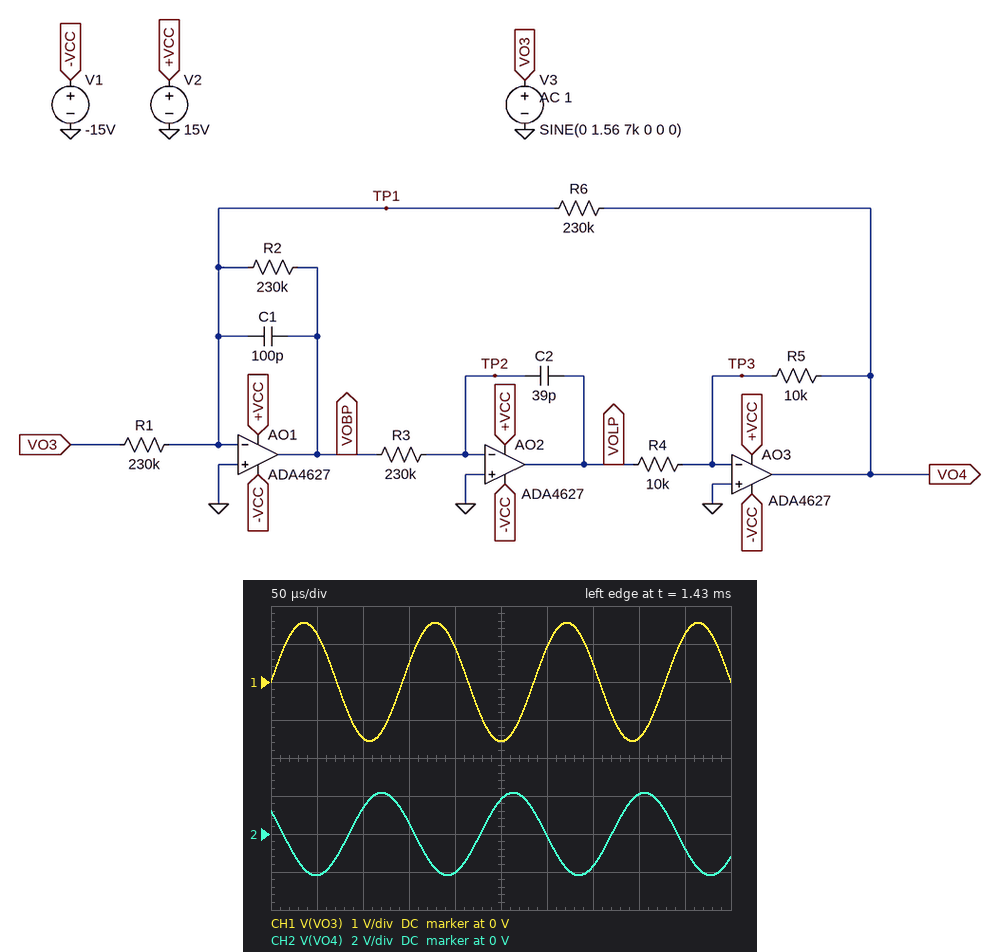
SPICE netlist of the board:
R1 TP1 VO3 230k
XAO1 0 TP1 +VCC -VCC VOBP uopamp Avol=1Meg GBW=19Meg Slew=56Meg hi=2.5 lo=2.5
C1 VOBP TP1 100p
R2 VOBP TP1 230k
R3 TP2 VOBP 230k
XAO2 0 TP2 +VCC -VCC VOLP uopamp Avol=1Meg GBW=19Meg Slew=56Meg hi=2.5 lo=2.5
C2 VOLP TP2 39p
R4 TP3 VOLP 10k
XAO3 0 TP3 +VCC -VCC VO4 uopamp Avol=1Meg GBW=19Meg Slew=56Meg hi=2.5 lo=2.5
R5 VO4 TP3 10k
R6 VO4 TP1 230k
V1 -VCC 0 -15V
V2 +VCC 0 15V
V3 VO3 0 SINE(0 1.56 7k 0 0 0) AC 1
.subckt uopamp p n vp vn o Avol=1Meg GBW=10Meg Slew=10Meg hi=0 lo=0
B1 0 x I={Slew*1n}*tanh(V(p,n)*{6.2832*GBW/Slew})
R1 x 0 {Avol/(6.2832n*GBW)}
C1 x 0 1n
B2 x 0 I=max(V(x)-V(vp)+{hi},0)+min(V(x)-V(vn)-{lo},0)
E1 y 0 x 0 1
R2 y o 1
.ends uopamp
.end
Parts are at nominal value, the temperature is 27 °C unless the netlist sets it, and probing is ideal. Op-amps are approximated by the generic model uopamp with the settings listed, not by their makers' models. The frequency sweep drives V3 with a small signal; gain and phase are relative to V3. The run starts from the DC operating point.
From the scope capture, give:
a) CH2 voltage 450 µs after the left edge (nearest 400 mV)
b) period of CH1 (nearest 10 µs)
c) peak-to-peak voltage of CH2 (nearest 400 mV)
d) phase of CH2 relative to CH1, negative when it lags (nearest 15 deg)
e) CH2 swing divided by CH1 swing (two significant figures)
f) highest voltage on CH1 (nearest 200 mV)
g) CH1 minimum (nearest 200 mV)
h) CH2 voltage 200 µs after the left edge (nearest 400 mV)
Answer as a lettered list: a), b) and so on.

a) -800 mV
b) 140 µs
c) 4.4 V
d) 150 deg
e) 1.4
f) 1.6 V
g) -1.6 V
h) -2.0 V
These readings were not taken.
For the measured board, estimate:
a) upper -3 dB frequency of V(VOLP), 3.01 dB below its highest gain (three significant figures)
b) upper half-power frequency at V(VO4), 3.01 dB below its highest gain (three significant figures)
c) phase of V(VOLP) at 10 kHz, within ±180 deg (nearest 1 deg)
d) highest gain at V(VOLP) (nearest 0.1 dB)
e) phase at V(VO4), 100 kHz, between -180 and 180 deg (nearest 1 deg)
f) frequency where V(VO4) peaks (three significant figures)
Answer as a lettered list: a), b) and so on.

a) 13.1 kHz
b) 13.1 kHz
c) -72 deg
d) 4.6 dB
e) 3 deg
f) 9.94 kHz
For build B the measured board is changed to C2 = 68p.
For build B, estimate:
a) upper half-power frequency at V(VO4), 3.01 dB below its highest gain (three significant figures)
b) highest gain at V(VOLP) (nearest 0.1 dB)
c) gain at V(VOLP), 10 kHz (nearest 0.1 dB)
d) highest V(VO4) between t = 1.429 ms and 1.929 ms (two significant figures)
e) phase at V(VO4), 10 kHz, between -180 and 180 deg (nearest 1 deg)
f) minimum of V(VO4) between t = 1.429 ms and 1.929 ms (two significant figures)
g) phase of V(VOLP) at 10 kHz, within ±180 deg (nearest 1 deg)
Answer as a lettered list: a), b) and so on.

a) 9.96 kHz
b) 2.5 dB
c) -0.6 dB
d) 2.1 V
e) 67 deg
f) -2.1 V
g) -113 deg
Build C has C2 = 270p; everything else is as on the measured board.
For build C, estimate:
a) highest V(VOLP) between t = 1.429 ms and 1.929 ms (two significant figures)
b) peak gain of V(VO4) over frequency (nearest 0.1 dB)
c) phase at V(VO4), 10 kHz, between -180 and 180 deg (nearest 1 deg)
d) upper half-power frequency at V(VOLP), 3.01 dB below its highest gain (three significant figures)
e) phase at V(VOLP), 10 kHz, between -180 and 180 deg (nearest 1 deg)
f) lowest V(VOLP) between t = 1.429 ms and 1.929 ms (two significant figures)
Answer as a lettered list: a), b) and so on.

a) 480 mV
b) 0 dB
c) 40 deg
d) 3.55 kHz
e) -140 deg
f) -480 mV
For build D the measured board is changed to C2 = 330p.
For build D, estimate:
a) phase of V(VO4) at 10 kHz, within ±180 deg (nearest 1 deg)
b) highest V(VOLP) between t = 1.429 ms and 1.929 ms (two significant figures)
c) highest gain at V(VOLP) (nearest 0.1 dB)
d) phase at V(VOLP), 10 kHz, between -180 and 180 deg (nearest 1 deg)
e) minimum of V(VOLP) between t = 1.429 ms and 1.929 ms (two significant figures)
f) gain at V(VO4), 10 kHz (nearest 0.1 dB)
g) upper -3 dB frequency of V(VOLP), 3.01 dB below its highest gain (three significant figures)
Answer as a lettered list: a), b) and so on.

a) 39 deg
b) 380 mV
c) 0 dB
d) -141 deg
e) -380 mV
f) -17.6 dB
g) 2.81 kHz
